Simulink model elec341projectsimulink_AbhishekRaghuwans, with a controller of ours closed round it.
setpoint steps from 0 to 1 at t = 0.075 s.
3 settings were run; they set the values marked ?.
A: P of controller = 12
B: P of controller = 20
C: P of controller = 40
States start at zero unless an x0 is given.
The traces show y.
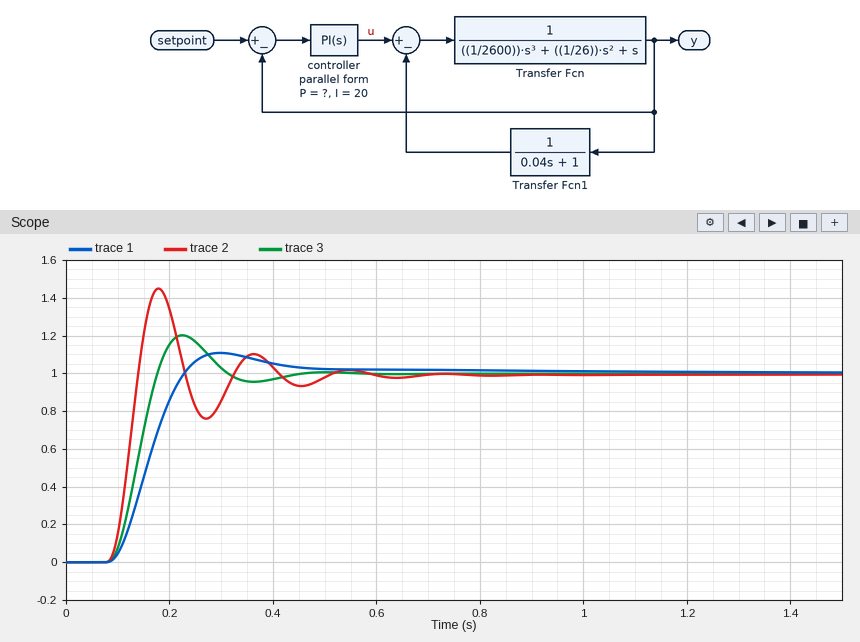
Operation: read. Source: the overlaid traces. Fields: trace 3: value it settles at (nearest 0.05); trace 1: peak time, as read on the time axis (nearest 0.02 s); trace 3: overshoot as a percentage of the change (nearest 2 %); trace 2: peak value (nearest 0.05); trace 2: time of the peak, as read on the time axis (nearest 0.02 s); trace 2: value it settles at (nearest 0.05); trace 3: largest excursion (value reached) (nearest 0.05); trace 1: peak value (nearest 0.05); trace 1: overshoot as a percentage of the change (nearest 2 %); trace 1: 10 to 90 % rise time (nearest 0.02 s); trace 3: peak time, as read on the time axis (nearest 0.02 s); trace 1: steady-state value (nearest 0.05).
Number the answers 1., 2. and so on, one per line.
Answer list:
1. 1.00
2. 0.30 s
3. 20 %
4. 1.45
5. 0.18 s
6. 1.00
7. 1.20
8. 1.10
9. 10 %
10. 0.10 s
11. 0.22 s
12. 1.00
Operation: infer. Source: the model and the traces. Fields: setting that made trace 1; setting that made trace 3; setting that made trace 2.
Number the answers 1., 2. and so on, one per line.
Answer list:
1. A
2. B
3. C
